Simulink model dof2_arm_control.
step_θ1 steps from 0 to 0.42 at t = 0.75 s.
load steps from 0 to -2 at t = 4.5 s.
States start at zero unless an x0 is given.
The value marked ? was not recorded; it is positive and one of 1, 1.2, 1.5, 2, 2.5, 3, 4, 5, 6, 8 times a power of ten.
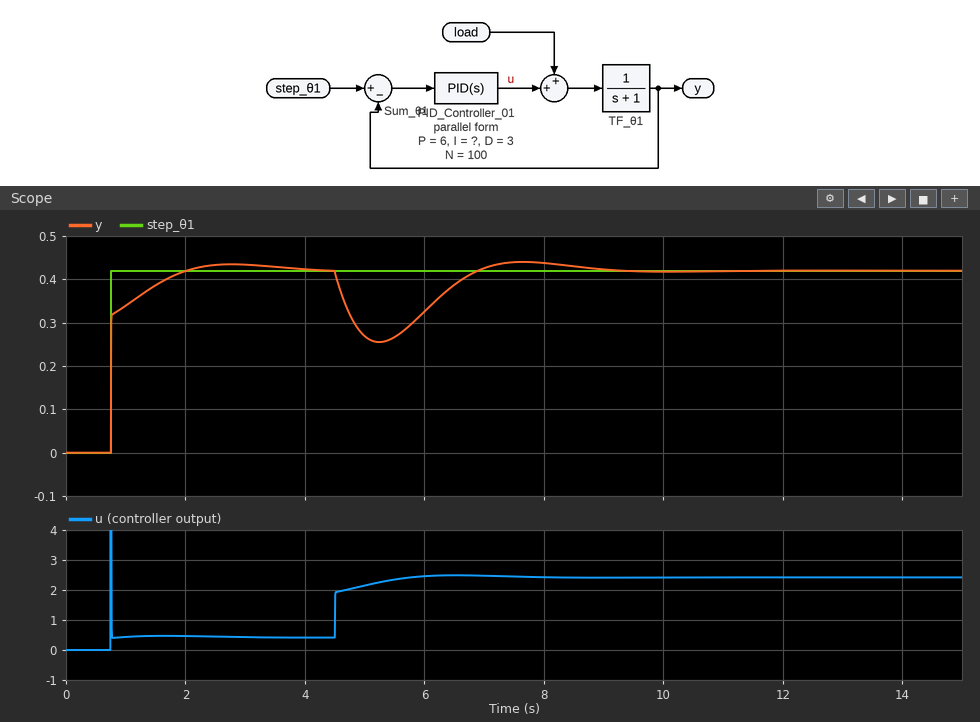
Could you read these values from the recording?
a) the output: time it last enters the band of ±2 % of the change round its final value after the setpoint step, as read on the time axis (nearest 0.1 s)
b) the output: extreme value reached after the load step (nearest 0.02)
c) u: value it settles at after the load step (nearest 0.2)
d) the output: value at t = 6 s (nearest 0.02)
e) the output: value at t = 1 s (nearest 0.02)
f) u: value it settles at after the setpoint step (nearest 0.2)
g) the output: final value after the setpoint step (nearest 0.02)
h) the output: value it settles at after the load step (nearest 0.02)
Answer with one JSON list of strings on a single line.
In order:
["3.5 s", "0.26", "2.4", "0.32", "0.34", "0.4", "0.42", "0.42"]
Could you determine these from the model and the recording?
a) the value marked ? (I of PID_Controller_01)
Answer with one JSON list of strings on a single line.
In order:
["10"]
